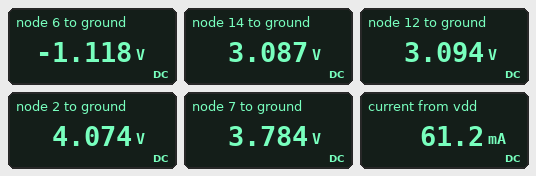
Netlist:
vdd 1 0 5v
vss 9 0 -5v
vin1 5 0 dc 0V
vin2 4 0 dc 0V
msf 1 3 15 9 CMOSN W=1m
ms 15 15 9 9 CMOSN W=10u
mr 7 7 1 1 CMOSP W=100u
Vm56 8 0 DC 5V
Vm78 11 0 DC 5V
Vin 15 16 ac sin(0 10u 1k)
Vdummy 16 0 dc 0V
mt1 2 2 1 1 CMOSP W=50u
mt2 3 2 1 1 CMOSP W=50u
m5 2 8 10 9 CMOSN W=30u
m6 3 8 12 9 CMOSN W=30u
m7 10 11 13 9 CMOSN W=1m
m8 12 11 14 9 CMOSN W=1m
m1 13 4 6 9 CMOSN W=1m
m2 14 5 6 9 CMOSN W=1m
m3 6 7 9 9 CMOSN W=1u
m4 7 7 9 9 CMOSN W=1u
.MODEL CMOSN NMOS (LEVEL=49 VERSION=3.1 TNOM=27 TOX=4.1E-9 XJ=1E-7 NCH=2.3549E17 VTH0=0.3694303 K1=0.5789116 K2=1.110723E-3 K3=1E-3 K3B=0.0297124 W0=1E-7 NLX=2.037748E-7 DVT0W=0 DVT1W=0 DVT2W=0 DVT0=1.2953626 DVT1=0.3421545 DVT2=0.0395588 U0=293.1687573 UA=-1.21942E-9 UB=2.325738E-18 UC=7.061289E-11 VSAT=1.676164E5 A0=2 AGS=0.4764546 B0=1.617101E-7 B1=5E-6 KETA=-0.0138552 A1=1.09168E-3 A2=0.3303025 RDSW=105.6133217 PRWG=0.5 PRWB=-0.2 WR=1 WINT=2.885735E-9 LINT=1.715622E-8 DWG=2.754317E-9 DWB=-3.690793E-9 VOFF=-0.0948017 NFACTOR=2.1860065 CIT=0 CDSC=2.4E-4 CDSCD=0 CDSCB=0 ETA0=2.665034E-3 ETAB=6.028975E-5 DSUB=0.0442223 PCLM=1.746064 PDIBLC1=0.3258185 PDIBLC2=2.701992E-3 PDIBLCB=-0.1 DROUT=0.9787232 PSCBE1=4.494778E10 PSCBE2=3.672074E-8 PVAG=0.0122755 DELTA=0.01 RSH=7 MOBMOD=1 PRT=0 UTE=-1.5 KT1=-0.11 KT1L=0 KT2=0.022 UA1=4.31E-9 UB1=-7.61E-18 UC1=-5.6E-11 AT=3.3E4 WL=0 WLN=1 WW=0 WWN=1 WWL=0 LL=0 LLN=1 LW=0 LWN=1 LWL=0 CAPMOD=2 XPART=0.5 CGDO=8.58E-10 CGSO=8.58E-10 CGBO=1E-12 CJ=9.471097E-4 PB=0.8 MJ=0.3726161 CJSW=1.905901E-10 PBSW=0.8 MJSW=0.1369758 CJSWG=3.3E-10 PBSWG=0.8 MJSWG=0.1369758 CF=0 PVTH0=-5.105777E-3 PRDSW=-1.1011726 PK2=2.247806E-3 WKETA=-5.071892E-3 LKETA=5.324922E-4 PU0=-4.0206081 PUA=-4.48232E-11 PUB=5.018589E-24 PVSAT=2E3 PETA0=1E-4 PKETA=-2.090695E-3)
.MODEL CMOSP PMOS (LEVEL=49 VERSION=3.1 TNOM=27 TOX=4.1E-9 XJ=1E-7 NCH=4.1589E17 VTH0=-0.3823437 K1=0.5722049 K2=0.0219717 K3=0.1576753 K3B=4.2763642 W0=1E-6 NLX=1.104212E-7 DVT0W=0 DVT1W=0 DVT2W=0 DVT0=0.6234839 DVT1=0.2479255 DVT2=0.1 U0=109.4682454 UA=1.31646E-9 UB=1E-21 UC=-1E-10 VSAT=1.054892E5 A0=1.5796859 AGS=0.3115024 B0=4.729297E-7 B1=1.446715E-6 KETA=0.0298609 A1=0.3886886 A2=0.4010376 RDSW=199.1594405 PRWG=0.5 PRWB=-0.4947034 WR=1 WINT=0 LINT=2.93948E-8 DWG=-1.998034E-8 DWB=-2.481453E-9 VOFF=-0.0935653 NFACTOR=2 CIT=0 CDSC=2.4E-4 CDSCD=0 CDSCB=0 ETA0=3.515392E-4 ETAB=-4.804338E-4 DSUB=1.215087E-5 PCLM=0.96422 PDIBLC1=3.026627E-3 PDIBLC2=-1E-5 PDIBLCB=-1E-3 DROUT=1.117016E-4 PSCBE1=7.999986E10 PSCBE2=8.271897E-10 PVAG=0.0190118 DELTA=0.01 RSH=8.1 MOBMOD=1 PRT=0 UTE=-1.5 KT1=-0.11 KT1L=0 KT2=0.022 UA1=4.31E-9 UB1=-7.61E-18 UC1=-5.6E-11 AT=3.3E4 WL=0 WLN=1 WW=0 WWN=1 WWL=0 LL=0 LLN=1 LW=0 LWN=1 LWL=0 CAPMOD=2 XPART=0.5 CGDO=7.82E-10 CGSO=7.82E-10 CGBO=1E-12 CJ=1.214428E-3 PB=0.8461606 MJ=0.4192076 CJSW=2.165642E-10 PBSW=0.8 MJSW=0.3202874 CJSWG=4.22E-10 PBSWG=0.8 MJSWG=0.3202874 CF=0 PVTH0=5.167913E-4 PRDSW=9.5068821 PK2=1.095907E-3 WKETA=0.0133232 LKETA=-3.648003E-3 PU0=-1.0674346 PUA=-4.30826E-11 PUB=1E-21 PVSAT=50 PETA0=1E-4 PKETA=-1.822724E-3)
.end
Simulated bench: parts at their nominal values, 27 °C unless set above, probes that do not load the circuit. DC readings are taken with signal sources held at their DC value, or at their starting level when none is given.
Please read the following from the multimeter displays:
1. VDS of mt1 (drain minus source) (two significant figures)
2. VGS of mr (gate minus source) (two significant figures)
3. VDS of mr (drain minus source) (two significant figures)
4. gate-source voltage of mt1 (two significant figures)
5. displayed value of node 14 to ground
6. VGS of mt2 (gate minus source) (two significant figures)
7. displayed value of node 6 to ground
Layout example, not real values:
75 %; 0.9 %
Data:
-930 mV; -1.2 V; -1.2 V; -930 mV; 3.087 V; -930 mV; -1.118 V
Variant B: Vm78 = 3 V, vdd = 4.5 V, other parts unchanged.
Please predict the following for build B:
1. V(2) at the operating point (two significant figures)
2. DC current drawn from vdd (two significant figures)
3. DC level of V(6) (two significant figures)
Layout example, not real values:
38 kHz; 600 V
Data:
3.6 V; 48 mA; -1.1 V
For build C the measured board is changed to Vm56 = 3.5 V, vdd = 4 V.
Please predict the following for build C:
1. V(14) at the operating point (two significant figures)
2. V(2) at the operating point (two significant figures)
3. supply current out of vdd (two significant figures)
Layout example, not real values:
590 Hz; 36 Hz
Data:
1.7 V; 3.0 V; 35 mA
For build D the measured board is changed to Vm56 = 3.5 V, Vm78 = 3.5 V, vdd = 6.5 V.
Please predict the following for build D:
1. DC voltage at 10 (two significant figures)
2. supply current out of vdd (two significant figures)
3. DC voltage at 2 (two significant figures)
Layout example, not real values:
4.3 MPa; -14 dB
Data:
1.8 V; 99 mA; 5.6 V
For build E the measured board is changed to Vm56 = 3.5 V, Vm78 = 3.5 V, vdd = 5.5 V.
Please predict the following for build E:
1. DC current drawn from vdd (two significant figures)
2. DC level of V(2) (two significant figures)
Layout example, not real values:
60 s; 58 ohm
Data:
74 mA; 4.6 V
